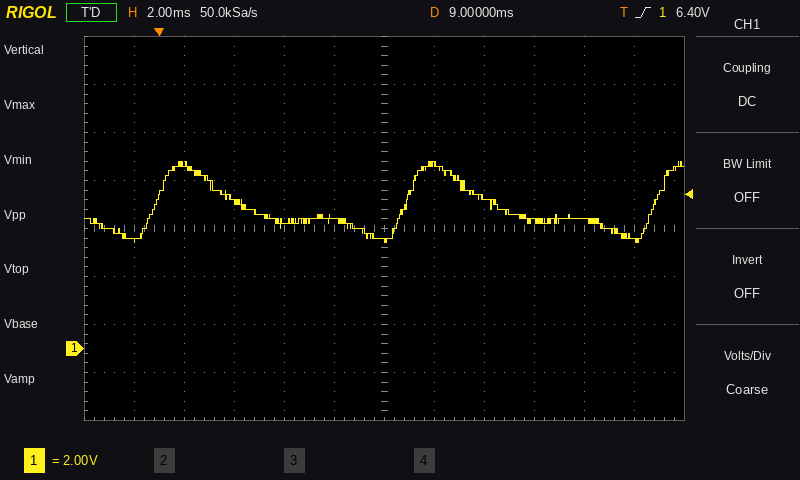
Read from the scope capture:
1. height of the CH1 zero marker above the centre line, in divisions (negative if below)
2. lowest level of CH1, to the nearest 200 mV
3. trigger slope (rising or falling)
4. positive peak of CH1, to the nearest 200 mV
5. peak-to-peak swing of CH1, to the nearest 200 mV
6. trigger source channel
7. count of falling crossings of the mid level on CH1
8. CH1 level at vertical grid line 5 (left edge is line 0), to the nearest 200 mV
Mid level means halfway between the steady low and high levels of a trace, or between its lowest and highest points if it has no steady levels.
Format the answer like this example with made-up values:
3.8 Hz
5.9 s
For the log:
-2.5 div
4.4 V
rising
7.8 V
3.4 V
CH1
2
5.4 V
